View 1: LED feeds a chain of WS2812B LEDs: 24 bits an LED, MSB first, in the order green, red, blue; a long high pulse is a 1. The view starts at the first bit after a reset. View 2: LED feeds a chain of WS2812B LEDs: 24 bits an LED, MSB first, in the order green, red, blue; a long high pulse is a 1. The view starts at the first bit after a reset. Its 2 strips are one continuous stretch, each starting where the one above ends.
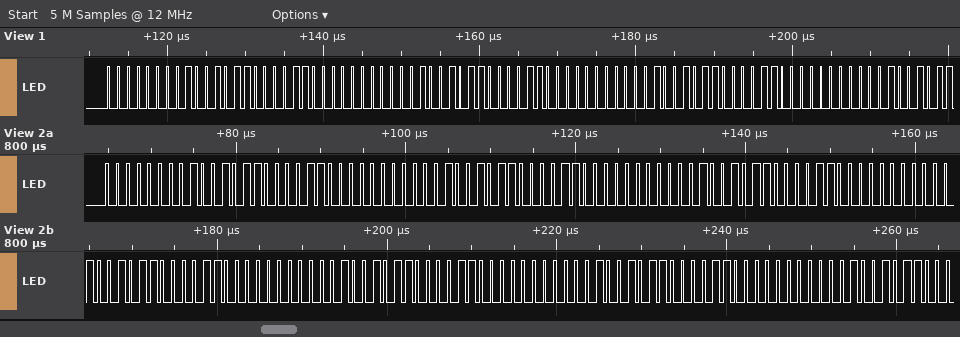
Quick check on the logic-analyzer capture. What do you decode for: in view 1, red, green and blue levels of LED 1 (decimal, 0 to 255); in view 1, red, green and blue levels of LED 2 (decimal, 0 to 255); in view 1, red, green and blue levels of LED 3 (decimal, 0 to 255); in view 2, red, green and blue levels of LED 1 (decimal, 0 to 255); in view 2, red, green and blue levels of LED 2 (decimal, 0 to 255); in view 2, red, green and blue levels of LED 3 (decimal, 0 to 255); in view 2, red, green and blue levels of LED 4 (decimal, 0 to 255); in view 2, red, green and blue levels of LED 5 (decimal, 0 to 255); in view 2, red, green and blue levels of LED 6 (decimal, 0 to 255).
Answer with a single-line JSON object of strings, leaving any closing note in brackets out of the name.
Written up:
{"in view 1, red, green and blue levels of LED 1": "150, 0, 24", "in view 1, red, green and blue levels of LED 2": "150, 0, 24", "in view 1, red, green and blue levels of LED 3": "150, 0, 24", "in view 2, red, green and blue levels of LED 1": "150, 0, 24", "in view 2, red, green and blue levels of LED 2": "150, 0, 24", "in view 2, red, green and blue levels of LED 3": "150, 0, 24", "in view 2, red, green and blue levels of LED 4": "150, 0, 24", "in view 2, red, green and blue levels of LED 5": "150, 0, 24", "in view 2, red, green and blue levels of LED 6": "150, 0, 24"}
